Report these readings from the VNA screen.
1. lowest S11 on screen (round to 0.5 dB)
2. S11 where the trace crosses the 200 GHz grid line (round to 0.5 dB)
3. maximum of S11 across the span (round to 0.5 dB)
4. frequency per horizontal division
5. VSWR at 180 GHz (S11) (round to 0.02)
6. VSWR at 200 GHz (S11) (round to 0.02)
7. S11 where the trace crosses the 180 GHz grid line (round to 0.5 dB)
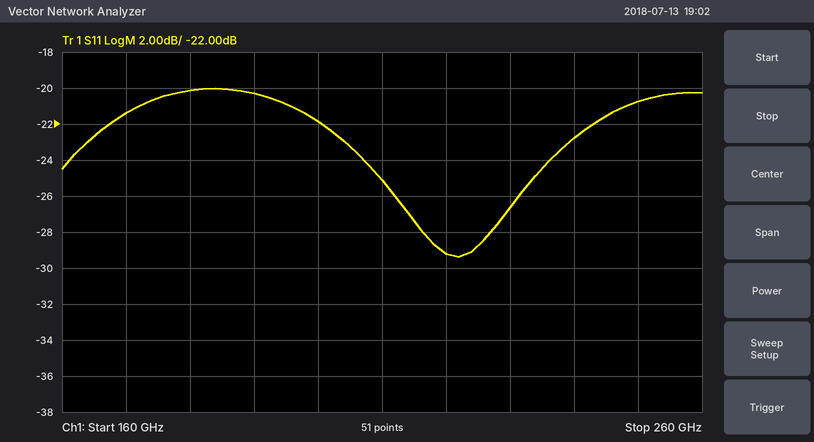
-29.5 dB
-22.0 dB
-20.0 dB
10 GHz
1.22
1.18
-20.0 dB
